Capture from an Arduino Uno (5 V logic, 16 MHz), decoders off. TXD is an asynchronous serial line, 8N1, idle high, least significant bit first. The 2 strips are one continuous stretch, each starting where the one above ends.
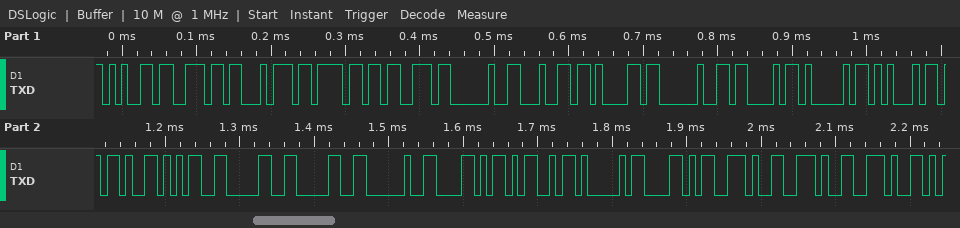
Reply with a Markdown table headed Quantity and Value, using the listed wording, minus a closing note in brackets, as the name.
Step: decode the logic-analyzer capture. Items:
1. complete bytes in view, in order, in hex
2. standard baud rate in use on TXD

| Quantity | Value |
|---|---|
| complete bytes in view, in order, in hex | 0x65 0x6E 0x74 0x6F 0x73 0x20 0x64 0x61 0x20 0x43 0x41 0x45 0x2D 0x35 0x30 0x30 0x20 0x58 0x4D 0x41 0x58 0x2E 0x2E 0x2E |
| standard baud rate in use on TXD | 115200 baud |
